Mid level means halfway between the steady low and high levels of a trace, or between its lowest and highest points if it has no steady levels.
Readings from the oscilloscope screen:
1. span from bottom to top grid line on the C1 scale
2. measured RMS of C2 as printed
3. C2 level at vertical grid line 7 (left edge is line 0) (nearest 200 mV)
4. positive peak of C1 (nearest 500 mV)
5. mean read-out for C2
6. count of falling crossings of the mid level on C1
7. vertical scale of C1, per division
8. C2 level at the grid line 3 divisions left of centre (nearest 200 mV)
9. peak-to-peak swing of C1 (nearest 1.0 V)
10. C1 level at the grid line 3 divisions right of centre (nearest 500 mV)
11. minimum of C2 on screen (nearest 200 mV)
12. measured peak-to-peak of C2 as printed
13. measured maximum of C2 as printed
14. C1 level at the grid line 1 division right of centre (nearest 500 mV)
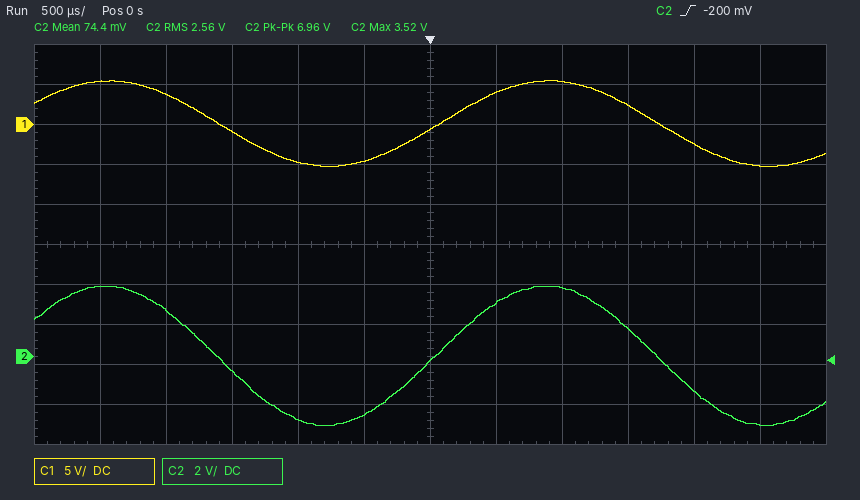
50 V
2.56 V
2.6 V
5.5 V
74.4 mV
2
5 V
-800 mV
11.0 V
2.5 V
-3.4 V
6.96 V
3.52 V
4.0 V
